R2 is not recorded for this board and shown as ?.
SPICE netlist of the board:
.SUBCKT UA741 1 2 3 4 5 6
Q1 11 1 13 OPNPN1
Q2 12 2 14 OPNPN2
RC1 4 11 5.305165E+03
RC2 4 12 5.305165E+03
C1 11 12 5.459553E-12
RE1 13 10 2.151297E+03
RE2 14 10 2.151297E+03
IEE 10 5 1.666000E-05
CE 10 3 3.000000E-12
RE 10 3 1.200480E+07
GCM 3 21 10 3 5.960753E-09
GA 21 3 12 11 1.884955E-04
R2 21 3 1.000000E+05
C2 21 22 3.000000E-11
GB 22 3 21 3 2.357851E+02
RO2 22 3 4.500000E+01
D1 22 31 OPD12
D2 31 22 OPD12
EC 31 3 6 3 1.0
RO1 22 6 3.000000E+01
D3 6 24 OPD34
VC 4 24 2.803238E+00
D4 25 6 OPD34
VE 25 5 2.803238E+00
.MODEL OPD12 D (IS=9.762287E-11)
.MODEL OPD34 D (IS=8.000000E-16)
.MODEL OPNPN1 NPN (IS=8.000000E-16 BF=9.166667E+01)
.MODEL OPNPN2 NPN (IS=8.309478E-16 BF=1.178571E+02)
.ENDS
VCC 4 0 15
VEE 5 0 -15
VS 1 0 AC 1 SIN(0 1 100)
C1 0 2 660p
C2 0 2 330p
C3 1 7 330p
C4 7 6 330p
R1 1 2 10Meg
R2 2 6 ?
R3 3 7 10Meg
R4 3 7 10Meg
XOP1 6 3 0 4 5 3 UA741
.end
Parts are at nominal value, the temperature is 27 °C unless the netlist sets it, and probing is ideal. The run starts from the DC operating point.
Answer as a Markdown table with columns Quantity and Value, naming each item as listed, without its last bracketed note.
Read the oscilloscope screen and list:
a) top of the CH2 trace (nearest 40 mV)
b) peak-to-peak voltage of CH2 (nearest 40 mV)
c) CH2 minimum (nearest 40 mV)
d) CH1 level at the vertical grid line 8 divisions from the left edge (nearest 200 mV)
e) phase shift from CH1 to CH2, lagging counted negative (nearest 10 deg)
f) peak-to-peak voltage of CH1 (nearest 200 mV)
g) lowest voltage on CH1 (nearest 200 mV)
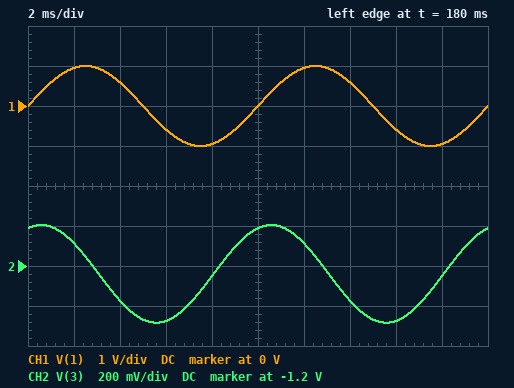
| Quantity | Value |
|---|---|
| top of the CH2 trace | -1.00 V |
| peak-to-peak voltage of CH2 | 480 mV |
| CH2 minimum | -1.48 V |
| CH1 level at the vertical grid line 8 divisions from the left edge | -600 mV |
| phase shift from CH1 to CH2, lagging counted negative | 70 deg |
| peak-to-peak voltage of CH1 | 2.0 V |
| lowest voltage on CH1 | -1.0 V |
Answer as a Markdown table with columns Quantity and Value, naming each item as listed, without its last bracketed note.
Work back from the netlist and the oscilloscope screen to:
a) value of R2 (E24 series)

| Quantity | Value |
|---|---|
| value of R2 | 3.9 MΩ |
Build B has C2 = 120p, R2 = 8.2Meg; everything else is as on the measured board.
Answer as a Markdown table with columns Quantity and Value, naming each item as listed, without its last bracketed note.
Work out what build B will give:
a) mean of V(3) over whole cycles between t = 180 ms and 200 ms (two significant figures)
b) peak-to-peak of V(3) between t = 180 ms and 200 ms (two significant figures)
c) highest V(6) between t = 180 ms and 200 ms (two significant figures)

| Quantity | Value |
|---|---|
| mean of V(3) over whole cycles between t = 180 ms and 200 ms | -1.6 V |
| peak-to-peak of V(3) between t = 180 ms and 200 ms | 1.1 V |
| highest V(6) between t = 180 ms and 200 ms | -1.1 V |
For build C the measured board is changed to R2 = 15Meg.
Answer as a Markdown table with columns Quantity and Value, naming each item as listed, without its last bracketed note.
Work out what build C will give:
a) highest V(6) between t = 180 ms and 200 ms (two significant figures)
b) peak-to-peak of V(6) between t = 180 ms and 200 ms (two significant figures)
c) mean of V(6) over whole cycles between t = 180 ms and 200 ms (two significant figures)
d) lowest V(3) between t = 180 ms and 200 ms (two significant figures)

| Quantity | Value |
|---|---|
| highest V(6) between t = 180 ms and 200 ms | -1.3 V |
| peak-to-peak of V(6) between t = 180 ms and 200 ms | 1.8 V |
| mean of V(6) over whole cycles between t = 180 ms and 200 ms | -2.2 V |
| lowest V(3) between t = 180 ms and 200 ms | -3.1 V |
